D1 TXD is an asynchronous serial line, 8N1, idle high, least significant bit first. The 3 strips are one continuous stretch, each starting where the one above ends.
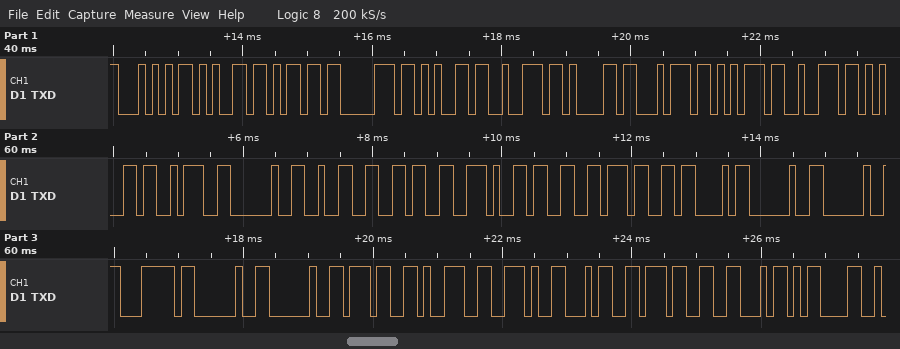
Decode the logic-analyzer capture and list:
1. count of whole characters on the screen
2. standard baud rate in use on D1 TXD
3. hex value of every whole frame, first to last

31
9600 baud
54 65 6D 70 65 72 61 74 75 72 65 3A 20 32 36 2E 33 37 43 20 20 7C 20 20 37 39 2E 34 37 46 0D
